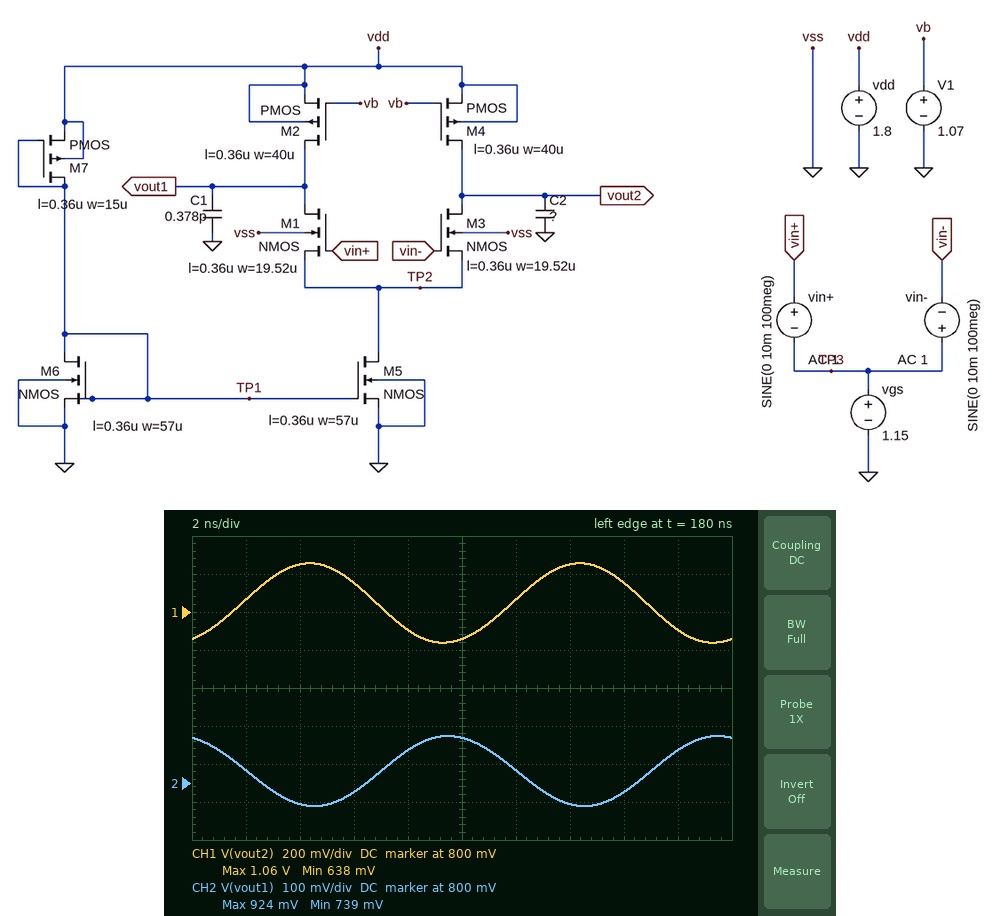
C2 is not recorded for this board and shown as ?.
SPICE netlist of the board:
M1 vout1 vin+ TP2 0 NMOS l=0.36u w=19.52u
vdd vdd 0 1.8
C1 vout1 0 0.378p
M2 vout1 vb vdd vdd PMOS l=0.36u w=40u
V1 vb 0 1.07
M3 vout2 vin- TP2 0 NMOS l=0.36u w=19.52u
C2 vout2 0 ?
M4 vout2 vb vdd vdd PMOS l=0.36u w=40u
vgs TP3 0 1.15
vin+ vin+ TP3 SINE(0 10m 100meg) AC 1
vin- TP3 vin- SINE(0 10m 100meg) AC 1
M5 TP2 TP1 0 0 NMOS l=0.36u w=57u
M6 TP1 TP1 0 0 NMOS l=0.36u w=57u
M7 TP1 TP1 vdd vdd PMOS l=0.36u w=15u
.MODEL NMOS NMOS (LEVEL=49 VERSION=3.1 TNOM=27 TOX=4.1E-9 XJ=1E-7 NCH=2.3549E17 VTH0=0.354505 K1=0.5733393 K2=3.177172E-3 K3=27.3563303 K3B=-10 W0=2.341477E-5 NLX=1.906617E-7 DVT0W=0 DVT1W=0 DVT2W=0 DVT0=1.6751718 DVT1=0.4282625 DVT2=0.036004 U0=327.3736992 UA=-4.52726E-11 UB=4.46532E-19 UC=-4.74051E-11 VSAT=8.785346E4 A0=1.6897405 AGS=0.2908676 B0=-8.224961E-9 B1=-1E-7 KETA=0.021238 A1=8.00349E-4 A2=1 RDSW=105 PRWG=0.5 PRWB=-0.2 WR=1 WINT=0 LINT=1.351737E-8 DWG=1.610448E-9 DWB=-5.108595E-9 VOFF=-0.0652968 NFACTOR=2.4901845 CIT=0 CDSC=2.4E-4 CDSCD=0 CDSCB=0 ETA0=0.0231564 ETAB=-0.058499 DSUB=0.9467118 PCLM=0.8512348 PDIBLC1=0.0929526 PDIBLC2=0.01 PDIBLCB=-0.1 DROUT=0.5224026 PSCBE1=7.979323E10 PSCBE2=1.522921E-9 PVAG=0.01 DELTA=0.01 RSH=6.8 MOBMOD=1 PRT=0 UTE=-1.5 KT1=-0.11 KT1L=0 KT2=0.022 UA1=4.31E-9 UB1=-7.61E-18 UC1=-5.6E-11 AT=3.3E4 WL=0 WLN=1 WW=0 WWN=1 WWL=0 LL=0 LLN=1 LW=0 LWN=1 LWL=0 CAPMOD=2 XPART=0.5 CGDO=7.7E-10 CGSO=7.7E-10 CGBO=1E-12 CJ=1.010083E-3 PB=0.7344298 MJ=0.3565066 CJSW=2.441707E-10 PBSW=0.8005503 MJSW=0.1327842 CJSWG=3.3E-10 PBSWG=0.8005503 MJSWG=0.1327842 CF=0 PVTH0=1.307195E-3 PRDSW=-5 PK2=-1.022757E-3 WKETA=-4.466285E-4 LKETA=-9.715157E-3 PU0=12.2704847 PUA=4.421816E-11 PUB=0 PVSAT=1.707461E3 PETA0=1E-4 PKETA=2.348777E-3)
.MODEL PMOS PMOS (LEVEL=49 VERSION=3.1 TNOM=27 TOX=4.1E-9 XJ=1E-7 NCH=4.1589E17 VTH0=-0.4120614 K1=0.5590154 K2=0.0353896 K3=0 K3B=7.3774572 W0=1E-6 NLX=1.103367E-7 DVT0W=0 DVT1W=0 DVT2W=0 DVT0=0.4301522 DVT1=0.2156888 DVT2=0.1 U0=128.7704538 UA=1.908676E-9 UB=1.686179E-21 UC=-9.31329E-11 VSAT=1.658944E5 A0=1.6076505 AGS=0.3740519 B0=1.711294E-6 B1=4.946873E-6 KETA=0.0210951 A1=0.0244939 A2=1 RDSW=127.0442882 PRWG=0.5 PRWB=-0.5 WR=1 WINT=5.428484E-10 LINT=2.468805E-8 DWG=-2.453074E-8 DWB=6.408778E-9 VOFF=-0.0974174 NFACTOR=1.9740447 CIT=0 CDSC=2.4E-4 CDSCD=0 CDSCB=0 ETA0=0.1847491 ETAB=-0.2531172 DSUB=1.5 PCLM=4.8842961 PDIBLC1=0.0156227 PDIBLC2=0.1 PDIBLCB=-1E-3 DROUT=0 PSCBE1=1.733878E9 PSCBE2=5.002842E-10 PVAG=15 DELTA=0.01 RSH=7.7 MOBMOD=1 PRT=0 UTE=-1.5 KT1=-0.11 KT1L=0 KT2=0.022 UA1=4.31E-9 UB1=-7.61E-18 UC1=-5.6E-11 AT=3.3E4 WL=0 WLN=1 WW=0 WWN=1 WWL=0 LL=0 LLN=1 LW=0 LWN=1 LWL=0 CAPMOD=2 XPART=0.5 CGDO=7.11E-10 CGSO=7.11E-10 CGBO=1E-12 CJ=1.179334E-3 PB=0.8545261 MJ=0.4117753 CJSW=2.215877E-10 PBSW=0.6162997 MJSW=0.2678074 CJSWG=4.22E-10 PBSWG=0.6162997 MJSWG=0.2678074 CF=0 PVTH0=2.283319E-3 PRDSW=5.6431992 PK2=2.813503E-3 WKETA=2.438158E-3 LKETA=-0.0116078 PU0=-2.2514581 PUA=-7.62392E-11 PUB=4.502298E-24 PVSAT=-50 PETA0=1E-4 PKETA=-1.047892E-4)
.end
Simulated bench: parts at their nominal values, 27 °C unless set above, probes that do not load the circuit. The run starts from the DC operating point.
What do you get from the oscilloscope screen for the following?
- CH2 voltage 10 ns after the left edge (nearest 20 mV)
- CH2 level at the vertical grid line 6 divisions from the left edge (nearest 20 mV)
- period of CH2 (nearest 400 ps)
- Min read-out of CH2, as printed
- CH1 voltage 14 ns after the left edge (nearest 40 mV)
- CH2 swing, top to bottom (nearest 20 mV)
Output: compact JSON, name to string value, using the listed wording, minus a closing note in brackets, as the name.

{"CH2 voltage 10 ns after the left edge": "920 mV", "CH2 level at the vertical grid line 6 divisions from the left edge": "840 mV", "period of CH2": "10.0 ns", "Min read-out of CH2, as printed": "739 mV", "CH1 voltage 14 ns after the left edge": "1.04 V", "CH2 swing, top to bottom": "180 mV"}
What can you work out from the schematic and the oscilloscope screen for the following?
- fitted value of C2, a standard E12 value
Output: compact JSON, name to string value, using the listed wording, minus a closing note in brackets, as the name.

{"fitted value of C2, a standard E12 value": "120 fF"}
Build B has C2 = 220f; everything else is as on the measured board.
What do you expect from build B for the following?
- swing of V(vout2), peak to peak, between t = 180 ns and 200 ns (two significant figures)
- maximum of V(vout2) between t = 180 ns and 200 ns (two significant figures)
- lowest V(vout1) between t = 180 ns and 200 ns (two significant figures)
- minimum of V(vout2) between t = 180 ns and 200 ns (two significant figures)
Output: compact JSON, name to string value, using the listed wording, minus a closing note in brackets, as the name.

{"swing of V(vout2), peak to peak, between t = 180 ns and 200 ns": "280 mV", "maximum of V(vout2) between t = 180 ns and 200 ns": "980 mV", "lowest V(vout1) between t = 180 ns and 200 ns": "740 mV", "minimum of V(vout2) between t = 180 ns and 200 ns": "700 mV"}
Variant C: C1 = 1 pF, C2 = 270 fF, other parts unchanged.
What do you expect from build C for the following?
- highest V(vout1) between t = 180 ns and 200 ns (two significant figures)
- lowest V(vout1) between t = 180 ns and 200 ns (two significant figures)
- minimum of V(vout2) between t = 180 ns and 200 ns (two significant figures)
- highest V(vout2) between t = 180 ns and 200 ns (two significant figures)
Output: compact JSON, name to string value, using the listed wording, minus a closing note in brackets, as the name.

{"highest V(vout1) between t = 180 ns and 200 ns": "880 mV", "lowest V(vout1) between t = 180 ns and 200 ns": "800 mV", "minimum of V(vout2) between t = 180 ns and 200 ns": "720 mV", "highest V(vout2) between t = 180 ns and 200 ns": "960 mV"}
